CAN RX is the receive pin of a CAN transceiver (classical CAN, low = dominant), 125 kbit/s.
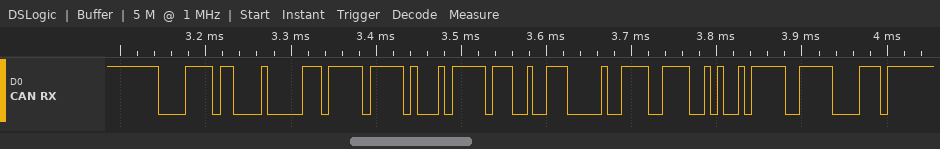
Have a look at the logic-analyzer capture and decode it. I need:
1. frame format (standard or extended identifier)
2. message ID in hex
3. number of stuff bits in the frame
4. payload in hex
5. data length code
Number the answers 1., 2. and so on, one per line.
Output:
1. standard
2. 0x0F6
3. 7
4. 37 FF 17 F9 38 0F 3C A5
5. 8
